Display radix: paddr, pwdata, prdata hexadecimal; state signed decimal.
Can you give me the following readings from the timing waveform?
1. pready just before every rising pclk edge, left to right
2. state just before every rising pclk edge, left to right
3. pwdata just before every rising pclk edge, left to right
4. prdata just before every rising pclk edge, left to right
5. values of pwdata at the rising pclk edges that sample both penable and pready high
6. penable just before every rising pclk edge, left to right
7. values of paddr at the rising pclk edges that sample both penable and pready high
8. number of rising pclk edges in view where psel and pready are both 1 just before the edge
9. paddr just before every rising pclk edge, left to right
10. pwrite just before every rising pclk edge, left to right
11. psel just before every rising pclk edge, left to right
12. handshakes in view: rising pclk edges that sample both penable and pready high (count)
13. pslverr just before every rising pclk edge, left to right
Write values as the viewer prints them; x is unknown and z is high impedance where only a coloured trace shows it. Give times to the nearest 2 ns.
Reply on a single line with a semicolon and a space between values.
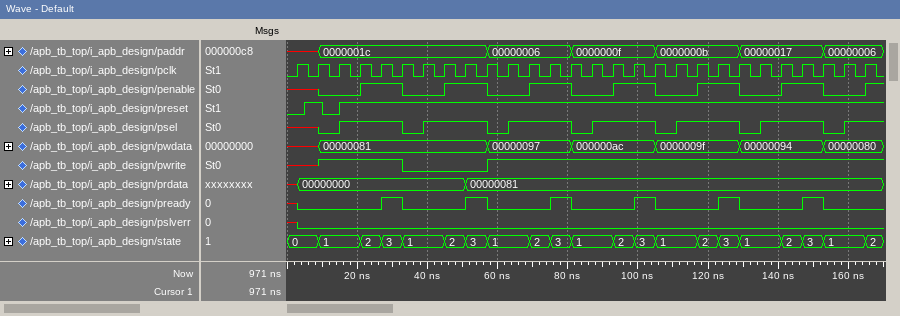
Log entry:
x 0 0 0 0 1 0 0 0 1 0 0 0 1 0 0 0 1 0 0 0 1 0 0 0 1 0 0; 0, 0, 1, 1, 2, 3, 1, 1, 2, 3, 1, 1, 2, 3, 1, 1, 2, 3, 1, 1, 2, 3, 1, 1, 2, 3, 1, 1; x, x, 00000081, 00000081, 00000081, 00000081, 00000081, 00000081, 00000081, 00000081, 00000097, 00000097, 00000097, 00000097, 000000ac, 000000ac, 000000ac, 000000ac, 0000009f, 0000009f, 0000009f, 0000009f, 00000094, 00000094, 00000094, 00000094, 00000080, 00000080; x, 00000000, 00000000, 00000000, 00000000, 00000000, 00000000, 00000000, 00000000, 00000081, 00000081, 00000081, 00000081, 00000081, 00000081, 00000081, 00000081, 00000081, 00000081, 00000081, 00000081, 00000081, 00000081, 00000081, 00000081, 00000081, 00000081, 00000081; 00000081, 00000081, 00000097, 000000ac, 0000009f, 00000094; x x 0 0 1 1 0 0 1 1 0 0 1 1 0 0 1 1 0 0 1 1 0 0 1 1 0 0; 0000001c, 0000001c, 00000006, 0000000f, 0000000b, 00000017; 6; x, x, 0000001c, 0000001c, 0000001c, 0000001c, 0000001c, 0000001c, 0000001c, 0000001c, 00000006, 00000006, 00000006, 00000006, 0000000f, 0000000f, 0000000f, 0000000f, 0000000b, 0000000b, 0000000b, 0000000b, 00000017, 00000017, 00000017, 00000017, 00000006, 00000006; x x 1 1 1 1 0 0 0 0 1 1 1 1 1 1 1 1 1 1 1 1 1 1 1 1 1 1; x x 0 1 1 1 0 1 1 1 0 1 1 1 0 1 1 1 0 1 1 1 0 1 1 1 0 1; 6; x 0 0 0 0 0 0 0 0 0 0 0 0 0 0 0 0 0 0 0 0 0 0 0 0 0 0 0
